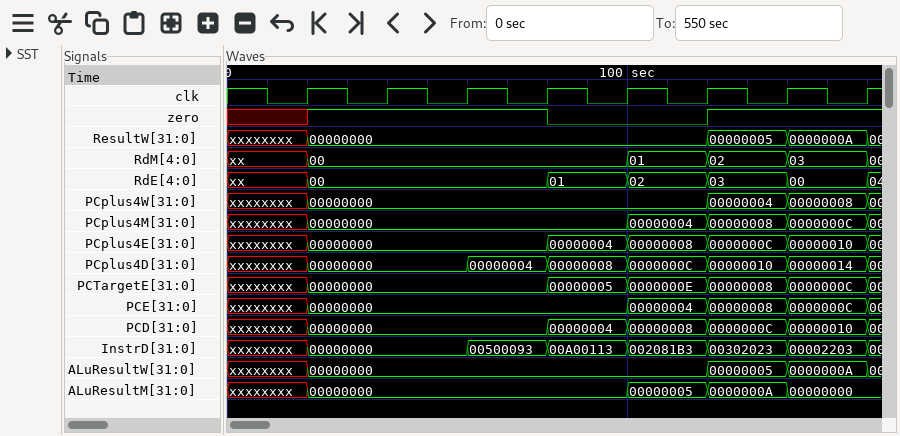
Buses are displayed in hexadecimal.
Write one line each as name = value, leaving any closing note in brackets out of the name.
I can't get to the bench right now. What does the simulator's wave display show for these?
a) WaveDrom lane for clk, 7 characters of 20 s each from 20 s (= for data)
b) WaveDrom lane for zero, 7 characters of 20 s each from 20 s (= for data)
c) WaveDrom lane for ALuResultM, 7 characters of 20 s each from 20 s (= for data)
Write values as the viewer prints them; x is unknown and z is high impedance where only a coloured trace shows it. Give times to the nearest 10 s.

WaveDrom lane for clk, 7 characters of 20 s each from 20 s = {name: 'clk', wave: 'p......'}
WaveDrom lane for zero, 7 characters of 20 s each from 20 s = {name: 'zero', wave: '1..0.1.'}
WaveDrom lane for ALuResultM, 7 characters of 20 s each from 20 s = {name: 'ALuResultM', wave: '=...===', data: '00000000 00000005 0000000A 00000000'}
